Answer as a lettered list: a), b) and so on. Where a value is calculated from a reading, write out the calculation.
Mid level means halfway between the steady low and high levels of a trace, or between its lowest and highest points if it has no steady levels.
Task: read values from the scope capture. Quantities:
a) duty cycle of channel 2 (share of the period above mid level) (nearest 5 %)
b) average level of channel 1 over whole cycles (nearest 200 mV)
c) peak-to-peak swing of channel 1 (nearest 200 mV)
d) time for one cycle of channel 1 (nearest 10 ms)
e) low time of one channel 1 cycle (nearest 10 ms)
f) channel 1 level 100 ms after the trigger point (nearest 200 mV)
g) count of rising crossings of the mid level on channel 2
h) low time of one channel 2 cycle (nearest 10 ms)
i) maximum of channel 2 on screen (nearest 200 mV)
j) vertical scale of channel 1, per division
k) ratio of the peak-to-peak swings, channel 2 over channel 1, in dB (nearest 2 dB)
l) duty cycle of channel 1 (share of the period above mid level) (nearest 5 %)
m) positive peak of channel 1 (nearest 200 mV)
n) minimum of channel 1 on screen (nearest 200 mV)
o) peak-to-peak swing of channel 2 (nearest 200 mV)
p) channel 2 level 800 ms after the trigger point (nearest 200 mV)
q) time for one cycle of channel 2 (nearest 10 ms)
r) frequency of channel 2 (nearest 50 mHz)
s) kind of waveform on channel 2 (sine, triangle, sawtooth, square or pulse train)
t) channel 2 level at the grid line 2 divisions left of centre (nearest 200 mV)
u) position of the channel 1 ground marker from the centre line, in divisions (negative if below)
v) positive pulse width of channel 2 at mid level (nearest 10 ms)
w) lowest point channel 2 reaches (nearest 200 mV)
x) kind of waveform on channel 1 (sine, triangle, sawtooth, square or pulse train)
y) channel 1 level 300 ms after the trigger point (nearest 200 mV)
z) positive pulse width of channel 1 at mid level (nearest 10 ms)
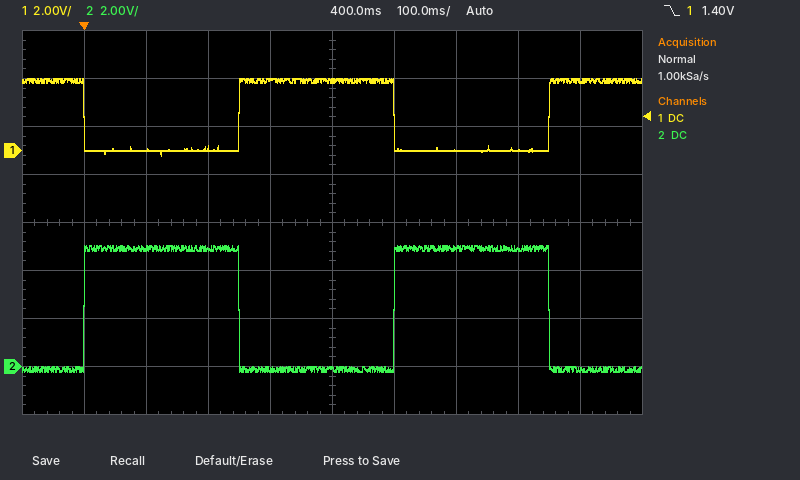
a) 250 ms / 500 ms ≈ 50 %
b) -200 mV + 0.5 × (3.0 V − (-200 mV)) ≈ 1.4 V
c) 3.0 V − (-200 mV) = 3.2 V
d) 500 ms
e) 250 ms
f) 0.0 V
g) 2
h) 250 ms
i) 5.0 V
j) 2 V
k) 20 log10(5.2 V / 3.2 V) ≈ 4 dB
l) 250 ms / 500 ms ≈ 50 %
m) 3.0 V
n) -200 mV
o) 5.0 V − (-200 mV) = 5.2 V
p) -200 mV
q) 500 ms
r) 1 / 500 ms ≈ 2.00 Hz
s) square
t) 5.0 V
u) +1.5 div
v) 250 ms
w) -200 mV
x) square
y) 3.0 V
z) 250 ms
